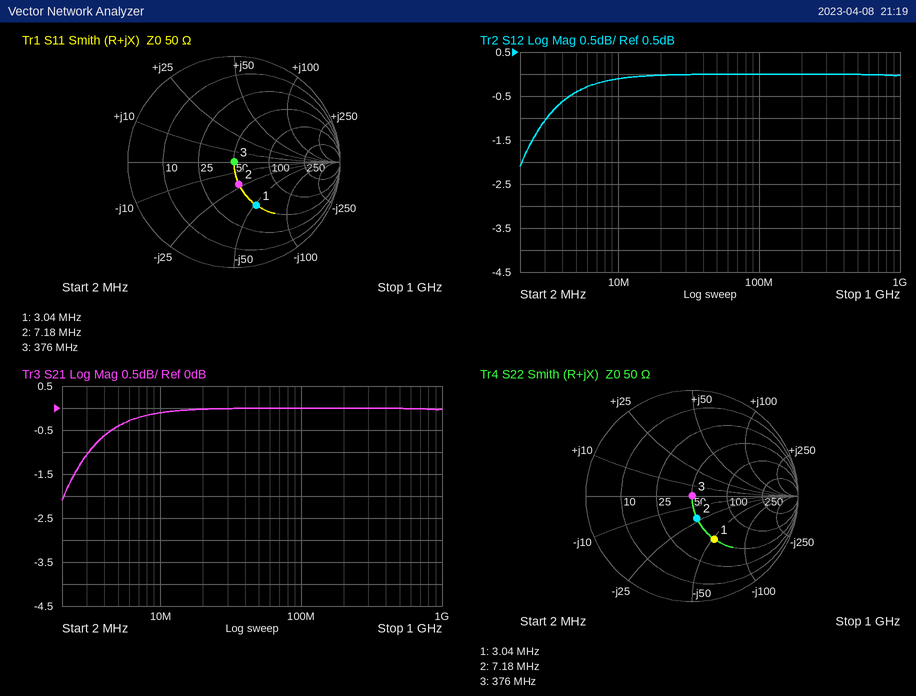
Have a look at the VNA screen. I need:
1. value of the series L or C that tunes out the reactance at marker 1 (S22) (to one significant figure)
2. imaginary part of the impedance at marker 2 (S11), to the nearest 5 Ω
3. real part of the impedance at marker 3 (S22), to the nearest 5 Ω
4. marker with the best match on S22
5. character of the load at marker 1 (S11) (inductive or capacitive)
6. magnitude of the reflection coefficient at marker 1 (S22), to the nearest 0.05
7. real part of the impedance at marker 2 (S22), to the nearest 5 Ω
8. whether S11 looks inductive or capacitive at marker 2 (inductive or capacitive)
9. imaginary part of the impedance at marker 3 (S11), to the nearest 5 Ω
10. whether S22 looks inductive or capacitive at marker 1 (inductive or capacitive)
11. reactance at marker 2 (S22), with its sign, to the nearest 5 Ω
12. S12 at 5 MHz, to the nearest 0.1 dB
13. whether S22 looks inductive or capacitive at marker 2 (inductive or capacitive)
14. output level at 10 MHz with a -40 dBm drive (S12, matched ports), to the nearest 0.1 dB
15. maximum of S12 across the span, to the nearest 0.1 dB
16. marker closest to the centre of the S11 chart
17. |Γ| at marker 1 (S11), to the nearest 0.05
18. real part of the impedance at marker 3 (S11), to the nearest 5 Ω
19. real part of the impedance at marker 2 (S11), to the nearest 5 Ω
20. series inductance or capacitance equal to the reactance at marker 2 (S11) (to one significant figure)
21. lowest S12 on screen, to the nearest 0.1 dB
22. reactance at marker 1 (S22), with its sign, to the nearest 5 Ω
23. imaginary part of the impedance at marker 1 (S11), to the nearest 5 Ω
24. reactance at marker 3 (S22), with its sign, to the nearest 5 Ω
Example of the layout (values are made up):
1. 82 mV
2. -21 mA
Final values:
1. 3 µH
2. -20 Ω
3. 50 Ω
4. marker 3
5. capacitive
6. 0.45
7. 50 Ω
8. capacitive
9. 0 Ω
10. capacitive
11. -20 Ω
12. -0.4 dB
13. capacitive
14. -40.1 dBm
15. 0.0 dB
16. marker 3
17. 0.45
18. 50 Ω
19. 50 Ω
20. 1 nF
21. -2.1 dB
22. -50 Ω
23. -50 Ω
24. 0 Ω
